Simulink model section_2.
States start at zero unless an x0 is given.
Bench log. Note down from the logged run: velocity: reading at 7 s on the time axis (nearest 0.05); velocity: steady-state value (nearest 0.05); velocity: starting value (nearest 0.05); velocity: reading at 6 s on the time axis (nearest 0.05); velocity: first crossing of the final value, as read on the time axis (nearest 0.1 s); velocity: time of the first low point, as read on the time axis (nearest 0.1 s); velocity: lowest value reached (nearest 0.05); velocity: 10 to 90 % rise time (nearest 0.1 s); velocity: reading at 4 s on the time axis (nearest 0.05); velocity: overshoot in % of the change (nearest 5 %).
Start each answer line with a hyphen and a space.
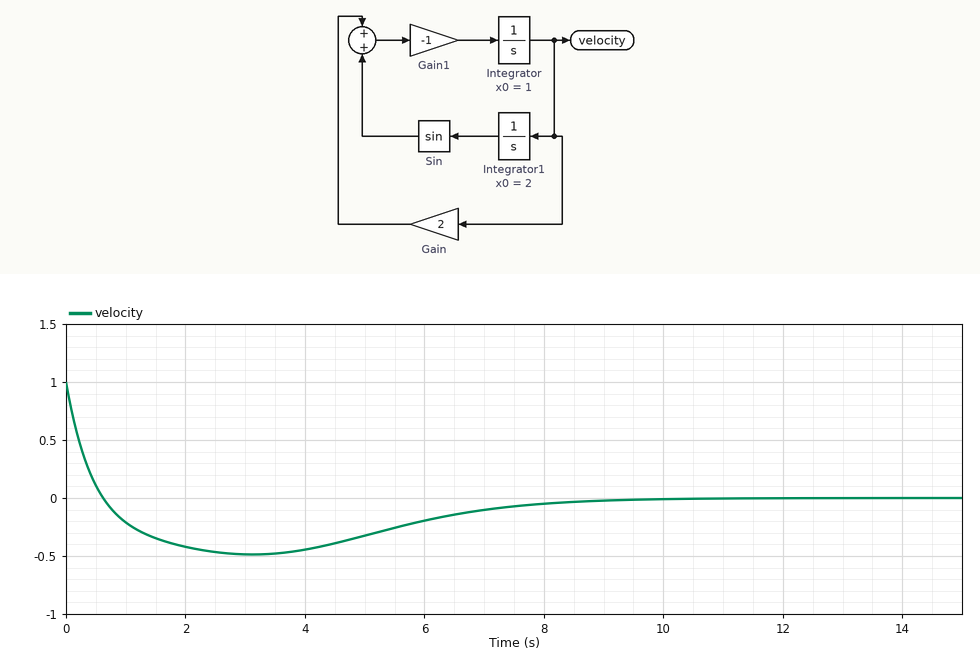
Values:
- -0.10
- 0.00
- 1.00
- -0.20
- 0.6 s
- 3.1 s
- -0.50
- 0.5 s
- -0.45
- 50 %
